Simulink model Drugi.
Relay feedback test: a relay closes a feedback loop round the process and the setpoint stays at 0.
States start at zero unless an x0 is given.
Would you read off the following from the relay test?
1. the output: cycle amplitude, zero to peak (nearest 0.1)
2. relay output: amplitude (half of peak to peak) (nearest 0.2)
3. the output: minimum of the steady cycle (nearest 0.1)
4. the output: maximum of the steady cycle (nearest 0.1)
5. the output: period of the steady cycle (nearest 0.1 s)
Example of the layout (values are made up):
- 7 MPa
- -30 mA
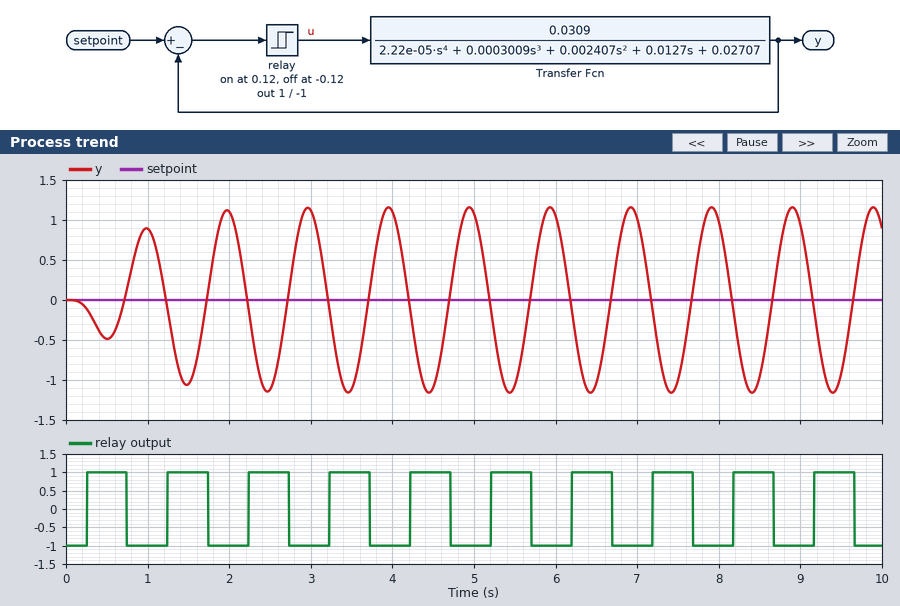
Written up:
- 1.2
- 1.0
- -1.2
- 1.2
- 1.0 s
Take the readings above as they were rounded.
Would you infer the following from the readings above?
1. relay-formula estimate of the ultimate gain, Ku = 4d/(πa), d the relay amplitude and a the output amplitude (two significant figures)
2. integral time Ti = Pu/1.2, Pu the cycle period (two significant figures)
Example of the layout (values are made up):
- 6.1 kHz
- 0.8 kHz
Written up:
- 1.1
- 0.83 s
